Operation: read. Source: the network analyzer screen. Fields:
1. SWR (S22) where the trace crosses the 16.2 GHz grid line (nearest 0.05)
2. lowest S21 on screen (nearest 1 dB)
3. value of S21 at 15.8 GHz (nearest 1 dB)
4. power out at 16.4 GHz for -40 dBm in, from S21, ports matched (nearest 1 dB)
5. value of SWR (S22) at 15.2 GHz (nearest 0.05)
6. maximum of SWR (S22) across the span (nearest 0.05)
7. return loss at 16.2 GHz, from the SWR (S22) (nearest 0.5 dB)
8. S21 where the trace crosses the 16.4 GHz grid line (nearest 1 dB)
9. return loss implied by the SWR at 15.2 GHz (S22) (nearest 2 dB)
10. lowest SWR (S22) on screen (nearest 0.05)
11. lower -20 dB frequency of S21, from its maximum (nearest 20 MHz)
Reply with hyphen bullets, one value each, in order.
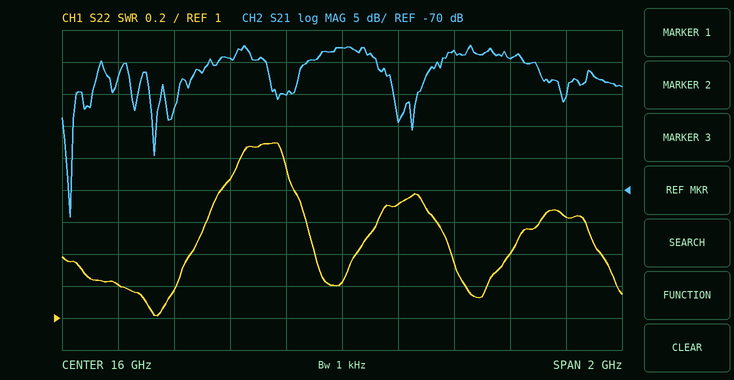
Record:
- 1.70
- -74 dB
- -55 dB
- -88 dBm
- 1.20
- 2.10
- 11.5 dB
- -48 dB
- 20 dB
- 1.00
- 15.04 GHz
